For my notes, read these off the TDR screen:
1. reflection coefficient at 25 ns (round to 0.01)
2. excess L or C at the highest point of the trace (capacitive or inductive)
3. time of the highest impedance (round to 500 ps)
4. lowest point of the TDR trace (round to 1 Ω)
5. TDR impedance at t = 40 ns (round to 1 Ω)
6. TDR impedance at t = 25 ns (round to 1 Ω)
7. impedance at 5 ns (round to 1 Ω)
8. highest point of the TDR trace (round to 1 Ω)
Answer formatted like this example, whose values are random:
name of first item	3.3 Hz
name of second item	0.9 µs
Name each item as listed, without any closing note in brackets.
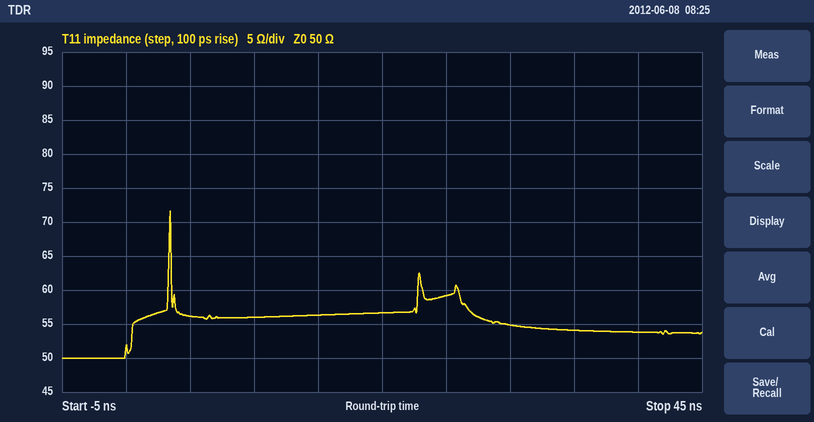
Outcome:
reflection coefficient at 25 ns	+0.08
excess L or C at the highest point of the trace	inductive
time of the highest impedance	3.5 ns
lowest point of the TDR trace	50 Ω
TDR impedance at t = 40 ns	54 Ω
TDR impedance at t = 25 ns	59 Ω
impedance at 5 ns	56 Ω
highest point of the TDR trace	72 Ω
